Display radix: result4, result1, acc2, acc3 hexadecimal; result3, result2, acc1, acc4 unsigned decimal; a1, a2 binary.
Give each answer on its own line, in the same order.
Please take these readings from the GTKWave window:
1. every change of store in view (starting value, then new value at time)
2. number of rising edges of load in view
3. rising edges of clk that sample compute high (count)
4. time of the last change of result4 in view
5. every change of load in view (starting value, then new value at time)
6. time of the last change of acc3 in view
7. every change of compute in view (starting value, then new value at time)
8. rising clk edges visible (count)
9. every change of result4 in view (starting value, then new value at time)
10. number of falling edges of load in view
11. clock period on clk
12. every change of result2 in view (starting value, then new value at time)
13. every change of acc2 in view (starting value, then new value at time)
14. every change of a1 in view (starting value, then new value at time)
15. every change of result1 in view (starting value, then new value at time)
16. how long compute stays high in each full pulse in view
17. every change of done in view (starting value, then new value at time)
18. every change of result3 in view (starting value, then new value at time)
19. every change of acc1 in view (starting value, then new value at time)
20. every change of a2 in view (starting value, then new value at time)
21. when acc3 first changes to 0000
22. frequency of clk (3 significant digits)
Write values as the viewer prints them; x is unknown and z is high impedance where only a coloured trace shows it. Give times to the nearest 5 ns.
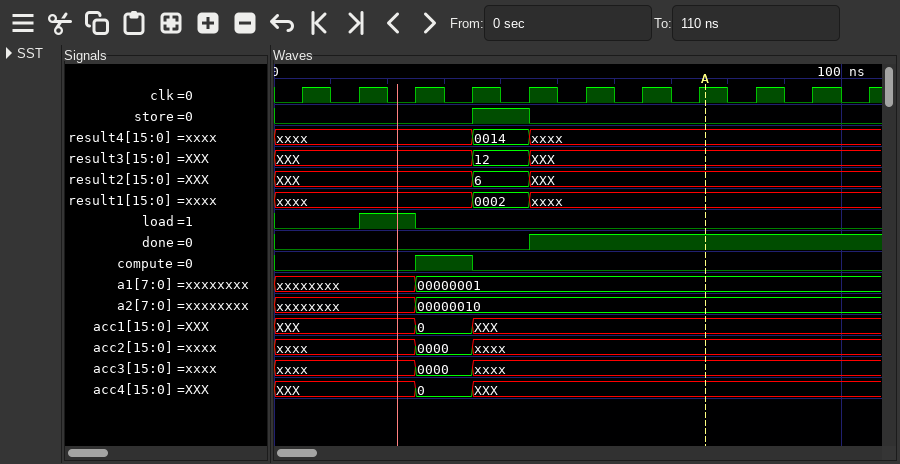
0, 1 at 35 ns, 0 at 45 ns
1
1
45 ns
0, 1 at 15 ns, 0 at 25 ns
35 ns
0, 1 at 25 ns, 0 at 35 ns
11
xxxx, 0014 at 35 ns, xxxx at 45 ns
1
10 ns
XXX, 6 at 35 ns, XXX at 45 ns
xxxx, 0000 at 25 ns, xxxx at 35 ns
xxxxxxxx, 00000001 at 25 ns
xxxx, 0002 at 35 ns, xxxx at 45 ns
10 ns
0, 1 at 45 ns
XXX, 12 at 35 ns, XXX at 45 ns
XXX, 0 at 25 ns, XXX at 35 ns
xxxxxxxx, 00000010 at 25 ns
25 ns
100 MHz
